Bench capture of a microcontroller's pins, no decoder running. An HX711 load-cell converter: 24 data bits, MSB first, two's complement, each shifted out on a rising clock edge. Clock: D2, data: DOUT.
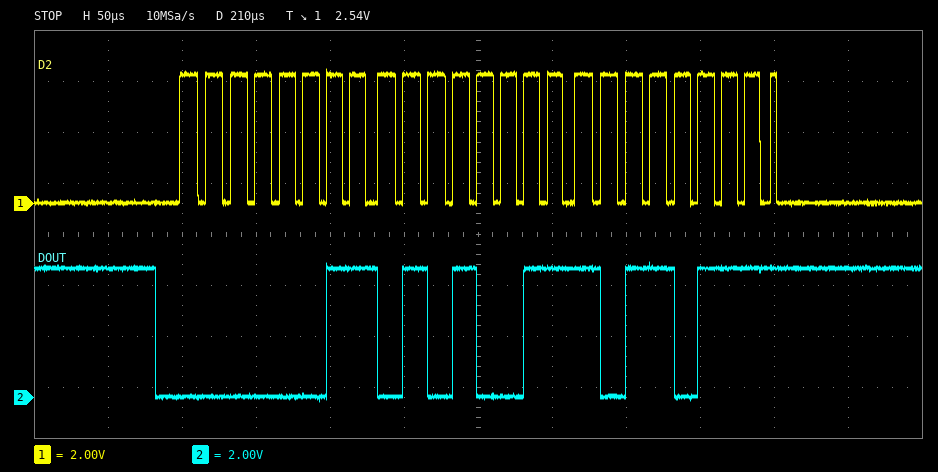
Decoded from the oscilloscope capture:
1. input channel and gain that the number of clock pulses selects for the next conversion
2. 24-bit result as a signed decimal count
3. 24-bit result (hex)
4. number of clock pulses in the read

channel A, gain 128
218039
0x0353B7
25
